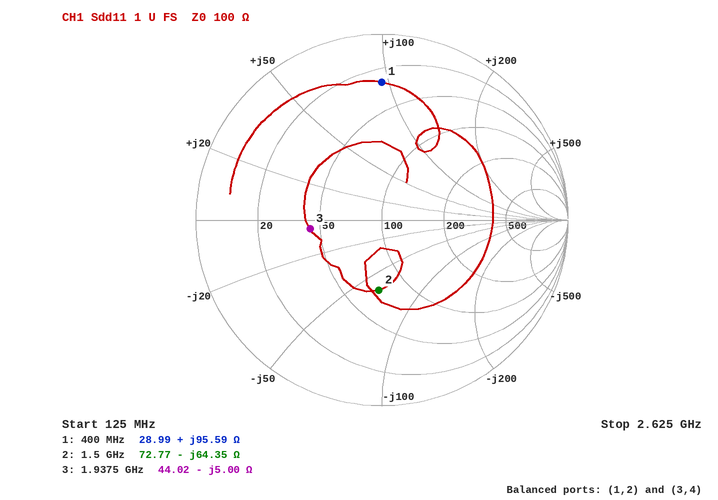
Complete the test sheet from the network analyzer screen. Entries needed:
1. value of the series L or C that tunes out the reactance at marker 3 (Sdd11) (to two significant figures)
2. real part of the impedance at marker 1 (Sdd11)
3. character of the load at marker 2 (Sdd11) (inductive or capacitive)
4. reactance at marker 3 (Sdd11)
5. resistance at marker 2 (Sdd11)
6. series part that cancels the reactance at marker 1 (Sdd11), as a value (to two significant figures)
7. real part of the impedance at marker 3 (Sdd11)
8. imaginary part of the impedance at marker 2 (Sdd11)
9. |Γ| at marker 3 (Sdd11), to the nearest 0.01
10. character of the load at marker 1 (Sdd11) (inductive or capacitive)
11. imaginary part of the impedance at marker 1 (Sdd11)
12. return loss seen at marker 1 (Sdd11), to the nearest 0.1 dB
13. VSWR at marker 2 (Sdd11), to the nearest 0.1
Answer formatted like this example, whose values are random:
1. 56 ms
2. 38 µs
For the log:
1. 410 pH
2. 28.99 Ω
3. capacitive
4. -5.00 Ω
5. 72.77 Ω
6. 4.2 pF
7. 44.02 Ω
8. -64.35 Ω
9. 0.39
10. inductive
11. +95.59 Ω
12. 2.6 dB
13. 2.2
